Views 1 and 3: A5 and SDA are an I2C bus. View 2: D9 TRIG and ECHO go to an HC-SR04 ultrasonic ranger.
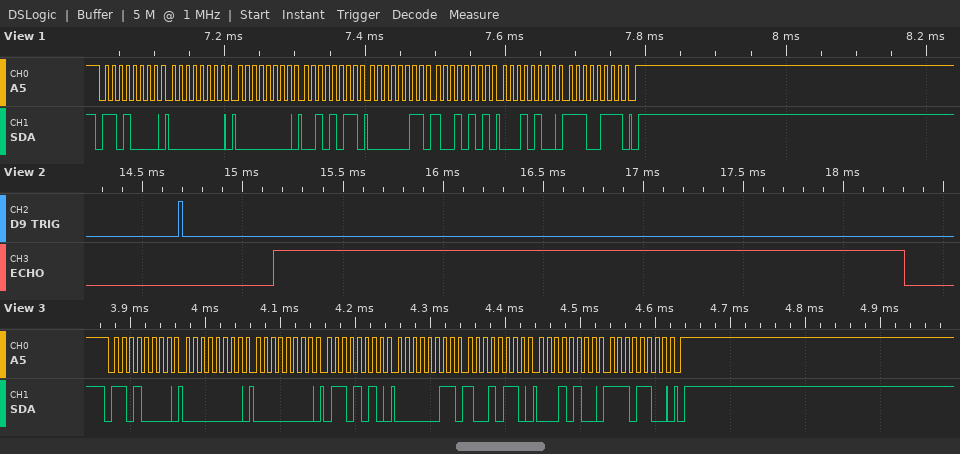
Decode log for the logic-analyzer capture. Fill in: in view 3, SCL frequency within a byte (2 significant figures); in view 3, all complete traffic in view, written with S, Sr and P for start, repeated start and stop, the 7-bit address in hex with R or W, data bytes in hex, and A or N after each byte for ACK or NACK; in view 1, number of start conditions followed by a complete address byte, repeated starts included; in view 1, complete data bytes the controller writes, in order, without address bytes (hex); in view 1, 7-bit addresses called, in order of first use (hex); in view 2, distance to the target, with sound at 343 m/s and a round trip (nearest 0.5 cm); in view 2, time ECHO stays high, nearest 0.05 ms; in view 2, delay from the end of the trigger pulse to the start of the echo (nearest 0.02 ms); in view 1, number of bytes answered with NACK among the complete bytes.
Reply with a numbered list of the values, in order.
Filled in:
1. 100 kHz
2. S 68W A 00 A 00 A 6A A 03 A 96 A 14 A EC A P
3. 1
4. 00 00 2B 03 95 14 E7
5. 0x68
6. 54 cm
7. 3.15 ms
8. 0.46 ms
9. 0
